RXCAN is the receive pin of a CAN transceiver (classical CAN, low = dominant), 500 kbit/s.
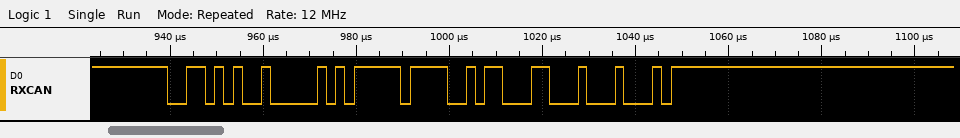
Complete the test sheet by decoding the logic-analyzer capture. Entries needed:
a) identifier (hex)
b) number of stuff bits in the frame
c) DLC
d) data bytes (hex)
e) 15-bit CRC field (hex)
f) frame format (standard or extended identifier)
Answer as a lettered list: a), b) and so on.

a) 0x352
b) 2
c) 2
d) FF 96
e) 0x1888
f) standard
